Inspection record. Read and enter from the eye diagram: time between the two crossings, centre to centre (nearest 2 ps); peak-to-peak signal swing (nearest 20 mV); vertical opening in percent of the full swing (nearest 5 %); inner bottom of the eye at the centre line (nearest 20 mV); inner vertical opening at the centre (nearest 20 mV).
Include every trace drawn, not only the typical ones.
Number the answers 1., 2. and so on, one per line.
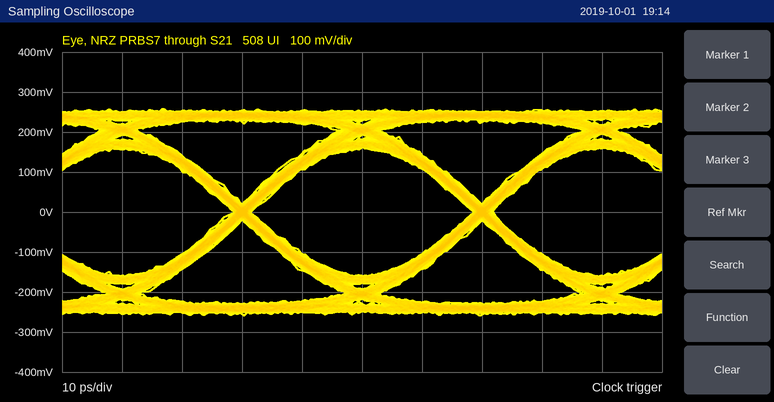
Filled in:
1. 40 ps
2. 520 mV
3. 60 %
4. -160 mV
5. 320 mV
